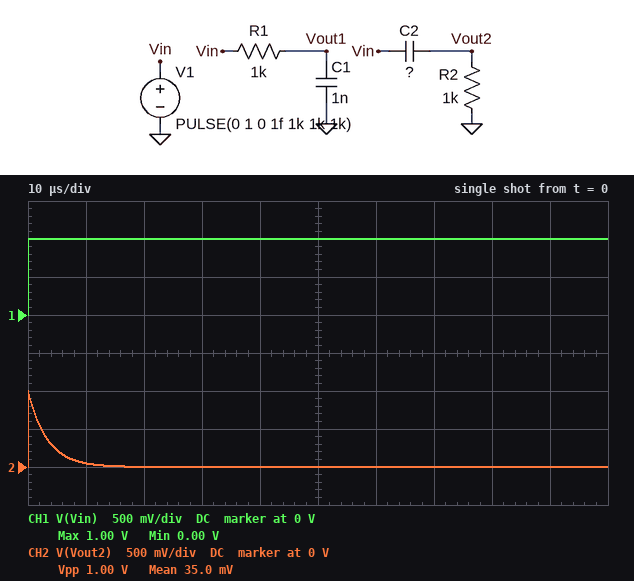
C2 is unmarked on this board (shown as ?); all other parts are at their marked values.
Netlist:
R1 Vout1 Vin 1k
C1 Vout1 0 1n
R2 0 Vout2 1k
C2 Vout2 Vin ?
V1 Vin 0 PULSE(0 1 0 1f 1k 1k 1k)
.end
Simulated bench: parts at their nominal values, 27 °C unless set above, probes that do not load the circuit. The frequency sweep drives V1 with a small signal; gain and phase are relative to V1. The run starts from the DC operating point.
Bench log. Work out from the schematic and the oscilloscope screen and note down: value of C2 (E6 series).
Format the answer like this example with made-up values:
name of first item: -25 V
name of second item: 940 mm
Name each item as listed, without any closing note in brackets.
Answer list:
value of C2: 3.3 nF
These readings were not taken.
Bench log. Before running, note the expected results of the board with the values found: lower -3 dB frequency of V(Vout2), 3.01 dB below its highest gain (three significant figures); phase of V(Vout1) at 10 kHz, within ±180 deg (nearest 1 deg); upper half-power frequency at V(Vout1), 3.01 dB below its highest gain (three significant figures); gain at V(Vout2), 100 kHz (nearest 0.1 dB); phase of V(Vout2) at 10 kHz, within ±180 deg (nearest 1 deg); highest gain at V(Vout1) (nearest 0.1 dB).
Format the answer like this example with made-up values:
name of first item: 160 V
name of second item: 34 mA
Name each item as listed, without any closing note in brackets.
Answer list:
lower -3 dB frequency of V(Vout2), 3.01 dB below its highest gain: 48.2 kHz
phase of V(Vout1) at 10 kHz, within ±180 deg: -4 deg
upper half-power frequency at V(Vout1), 3.01 dB below its highest gain: 159 kHz
gain at V(Vout2), 100 kHz: -0.9 dB
phase of V(Vout2) at 10 kHz, within ±180 deg: 78 deg
highest gain at V(Vout1): 0 dB
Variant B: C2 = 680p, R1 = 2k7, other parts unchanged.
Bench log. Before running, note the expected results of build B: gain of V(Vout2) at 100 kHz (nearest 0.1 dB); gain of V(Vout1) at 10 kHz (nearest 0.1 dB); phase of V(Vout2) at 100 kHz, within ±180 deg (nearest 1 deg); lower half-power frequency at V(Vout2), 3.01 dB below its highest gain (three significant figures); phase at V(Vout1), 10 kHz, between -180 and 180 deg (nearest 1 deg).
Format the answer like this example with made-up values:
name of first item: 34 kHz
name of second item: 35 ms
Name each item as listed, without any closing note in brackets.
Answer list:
gain of V(Vout2) at 100 kHz: -8.1 dB
gain of V(Vout1) at 10 kHz: -0.1 dB
phase of V(Vout2) at 100 kHz, within ±180 deg: 67 deg
lower half-power frequency at V(Vout2), 3.01 dB below its highest gain: 234 kHz
phase at V(Vout1), 10 kHz, between -180 and 180 deg: -10 deg
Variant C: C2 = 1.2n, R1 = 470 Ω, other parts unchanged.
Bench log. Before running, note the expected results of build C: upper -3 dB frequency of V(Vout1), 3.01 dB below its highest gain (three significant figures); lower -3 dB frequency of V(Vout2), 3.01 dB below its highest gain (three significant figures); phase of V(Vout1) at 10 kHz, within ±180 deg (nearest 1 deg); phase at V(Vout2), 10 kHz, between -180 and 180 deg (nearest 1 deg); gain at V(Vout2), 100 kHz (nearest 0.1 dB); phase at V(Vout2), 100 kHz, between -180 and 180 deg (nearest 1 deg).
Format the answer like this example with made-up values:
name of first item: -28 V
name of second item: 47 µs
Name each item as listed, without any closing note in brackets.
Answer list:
upper -3 dB frequency of V(Vout1), 3.01 dB below its highest gain: 339 kHz
lower -3 dB frequency of V(Vout2), 3.01 dB below its highest gain: 133 kHz
phase of V(Vout1) at 10 kHz, within ±180 deg: -2 deg
phase at V(Vout2), 10 kHz, between -180 and 180 deg: 86 deg
gain at V(Vout2), 100 kHz: -4.4 dB
phase at V(Vout2), 100 kHz, between -180 and 180 deg: 53 deg
